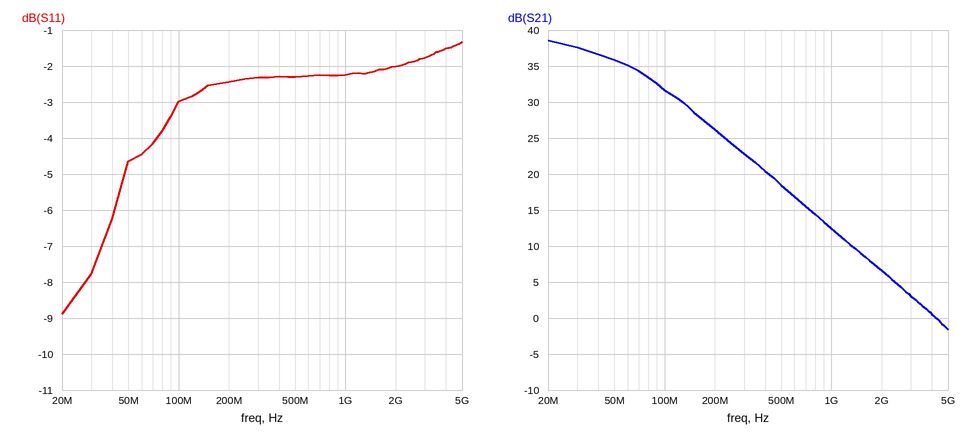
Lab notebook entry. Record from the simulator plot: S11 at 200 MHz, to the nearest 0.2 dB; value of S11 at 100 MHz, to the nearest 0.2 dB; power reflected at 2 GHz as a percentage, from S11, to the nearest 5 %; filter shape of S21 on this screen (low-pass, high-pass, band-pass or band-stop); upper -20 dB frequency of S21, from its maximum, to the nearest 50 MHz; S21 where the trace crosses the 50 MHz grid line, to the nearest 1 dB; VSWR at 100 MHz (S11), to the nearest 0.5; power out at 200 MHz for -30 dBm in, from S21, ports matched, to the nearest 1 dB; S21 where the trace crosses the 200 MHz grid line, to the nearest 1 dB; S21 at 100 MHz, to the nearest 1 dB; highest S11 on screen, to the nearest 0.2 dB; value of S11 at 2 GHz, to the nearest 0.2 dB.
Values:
-2.4 dB
-3.0 dB
65 %
low-pass
500 MHz
36 dB
6.0
-4 dBm
26 dB
32 dB
-1.4 dB
-2.0 dB
